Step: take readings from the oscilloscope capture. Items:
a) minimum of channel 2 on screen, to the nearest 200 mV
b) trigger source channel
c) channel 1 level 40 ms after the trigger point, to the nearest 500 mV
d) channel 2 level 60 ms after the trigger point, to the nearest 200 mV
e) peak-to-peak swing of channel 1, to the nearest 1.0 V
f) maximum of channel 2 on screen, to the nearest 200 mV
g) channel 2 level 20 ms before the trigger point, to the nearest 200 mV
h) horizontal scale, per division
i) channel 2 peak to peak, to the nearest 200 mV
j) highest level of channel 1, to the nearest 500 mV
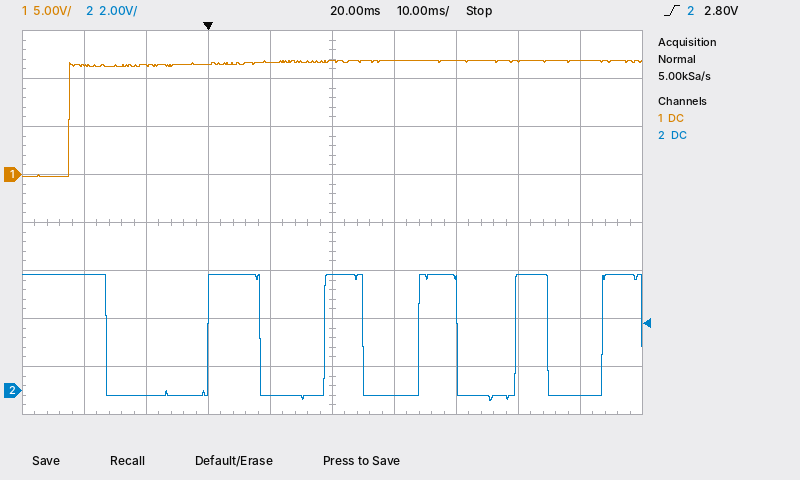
-400 mV
channel 2
12.0 V
-200 mV
12.0 V
4.8 V
4.8 V
10 ms
5.2 V
12.0 V
